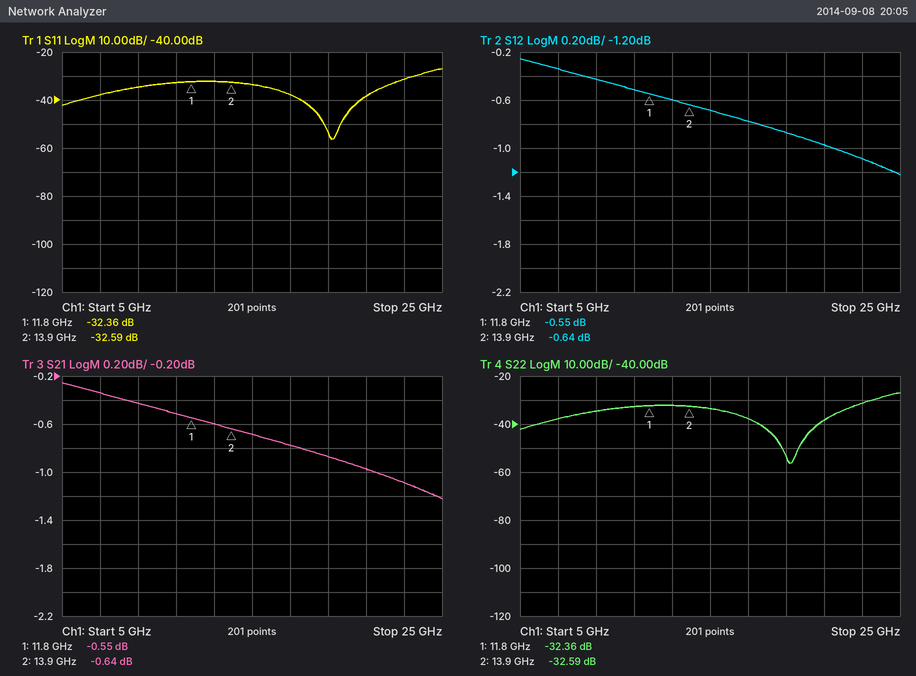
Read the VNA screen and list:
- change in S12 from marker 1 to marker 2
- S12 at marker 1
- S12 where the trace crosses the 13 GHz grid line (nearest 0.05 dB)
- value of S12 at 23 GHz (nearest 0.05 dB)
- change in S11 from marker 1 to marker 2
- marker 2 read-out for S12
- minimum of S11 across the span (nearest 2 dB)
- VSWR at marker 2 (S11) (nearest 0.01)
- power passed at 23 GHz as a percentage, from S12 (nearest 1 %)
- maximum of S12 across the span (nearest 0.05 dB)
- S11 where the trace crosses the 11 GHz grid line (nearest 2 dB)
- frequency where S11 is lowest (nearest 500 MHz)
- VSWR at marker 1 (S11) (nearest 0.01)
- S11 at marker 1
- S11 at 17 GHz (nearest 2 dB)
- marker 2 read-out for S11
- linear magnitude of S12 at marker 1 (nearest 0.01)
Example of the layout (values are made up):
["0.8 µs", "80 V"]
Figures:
["-0.09 dB", "-0.55 dB", "-0.60 dB", "-1.10 dB", "-0.23 dB", "-0.64 dB", "-56 dB", "1.05", "78 %", "-0.25 dB", "-32 dB", "19.0 GHz", "1.05", "-32.36 dB", "-38 dB", "-32.59 dB", "0.94"]
